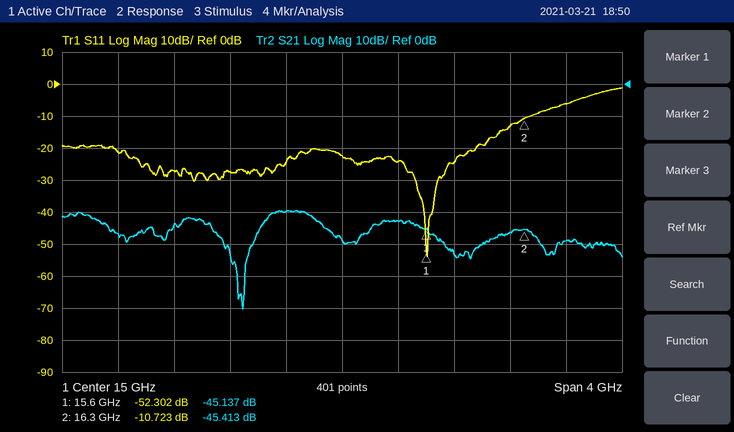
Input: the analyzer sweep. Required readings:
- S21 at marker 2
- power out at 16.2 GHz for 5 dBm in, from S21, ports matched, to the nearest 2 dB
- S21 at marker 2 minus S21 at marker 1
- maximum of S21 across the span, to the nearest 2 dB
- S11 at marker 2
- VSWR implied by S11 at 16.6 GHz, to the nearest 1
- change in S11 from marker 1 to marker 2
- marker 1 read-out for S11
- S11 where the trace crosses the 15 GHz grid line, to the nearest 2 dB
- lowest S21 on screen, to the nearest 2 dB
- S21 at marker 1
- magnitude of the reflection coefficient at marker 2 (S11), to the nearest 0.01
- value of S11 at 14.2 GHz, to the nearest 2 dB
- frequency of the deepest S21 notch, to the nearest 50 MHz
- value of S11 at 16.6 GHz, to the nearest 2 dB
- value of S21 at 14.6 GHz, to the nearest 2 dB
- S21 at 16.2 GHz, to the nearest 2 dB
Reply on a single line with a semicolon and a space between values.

-45.413 dB; -42 dBm; -0.276 dB; -40 dB; -10.723 dB; 3; 41.579 dB; -52.302 dB; -22 dB; -70 dB; -45.137 dB; 0.29; -28 dB; 14.30 GHz; -6 dB; -40 dB; -46 dB
